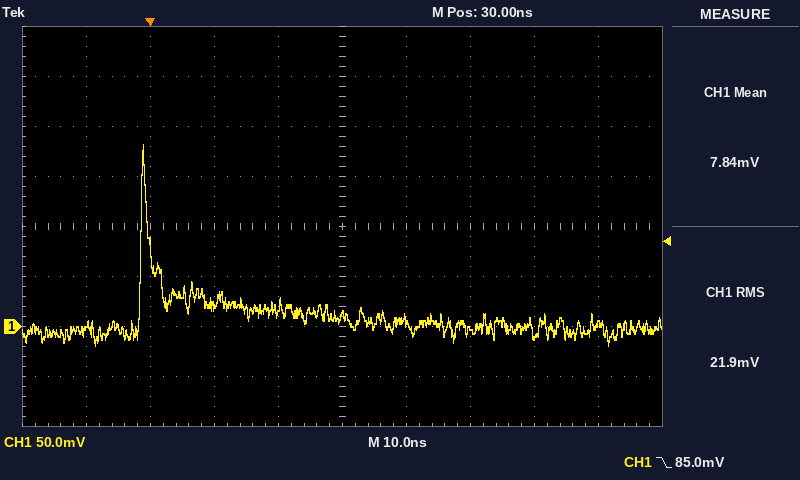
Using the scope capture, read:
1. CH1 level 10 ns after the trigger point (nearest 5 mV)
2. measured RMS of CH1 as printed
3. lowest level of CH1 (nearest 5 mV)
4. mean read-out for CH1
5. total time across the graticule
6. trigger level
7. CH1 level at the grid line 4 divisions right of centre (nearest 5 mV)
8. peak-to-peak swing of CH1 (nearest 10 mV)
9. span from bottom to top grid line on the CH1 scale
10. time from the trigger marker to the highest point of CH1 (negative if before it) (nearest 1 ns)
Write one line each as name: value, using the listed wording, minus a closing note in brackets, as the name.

CH1 level 10 ns after the trigger point: 20 mV
measured RMS of CH1 as printed: 21.9 mV
lowest level of CH1: -20 mV
mean read-out for CH1: 7.84 mV
total time across the graticule: 100 ns
trigger level: 85.0 mV
CH1 level at the grid line 4 divisions right of centre: 0 mV
peak-to-peak swing of CH1: 200 mV
span from bottom to top grid line on the CH1 scale: 400 mV
time from the trigger marker to the highest point of CH1 (negative if before it): -1 ns
